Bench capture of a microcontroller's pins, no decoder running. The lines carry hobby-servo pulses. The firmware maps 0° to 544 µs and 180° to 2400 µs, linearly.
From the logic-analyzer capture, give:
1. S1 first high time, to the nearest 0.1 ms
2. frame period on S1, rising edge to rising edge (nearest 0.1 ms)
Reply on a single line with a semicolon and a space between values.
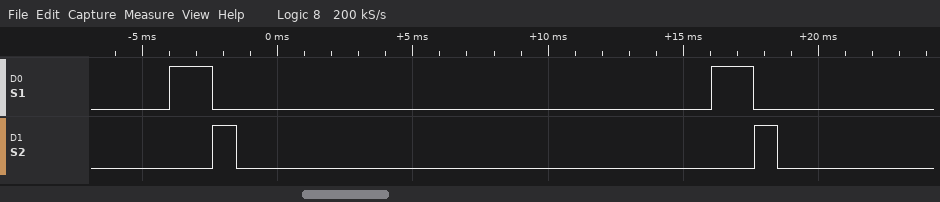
1.6 ms; 20.0 ms
